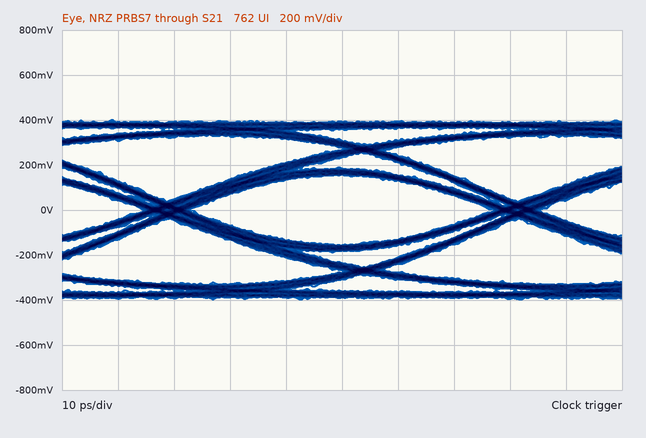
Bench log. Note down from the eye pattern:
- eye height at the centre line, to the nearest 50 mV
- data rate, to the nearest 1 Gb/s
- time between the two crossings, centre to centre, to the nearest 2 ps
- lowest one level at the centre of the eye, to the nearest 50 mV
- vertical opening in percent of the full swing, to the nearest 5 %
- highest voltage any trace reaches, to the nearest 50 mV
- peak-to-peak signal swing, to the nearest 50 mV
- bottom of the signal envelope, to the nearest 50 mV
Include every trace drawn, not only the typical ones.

300 mV
16 Gb/s
62 ps
150 mV
40 %
400 mV
800 mV
-400 mV
